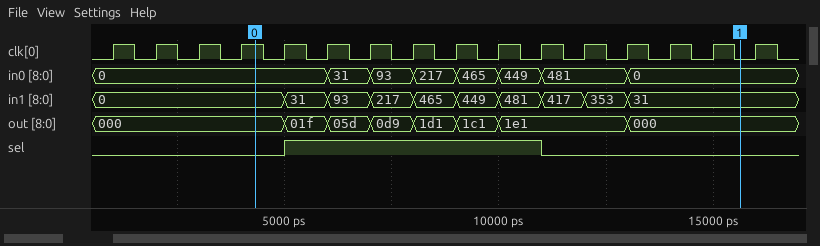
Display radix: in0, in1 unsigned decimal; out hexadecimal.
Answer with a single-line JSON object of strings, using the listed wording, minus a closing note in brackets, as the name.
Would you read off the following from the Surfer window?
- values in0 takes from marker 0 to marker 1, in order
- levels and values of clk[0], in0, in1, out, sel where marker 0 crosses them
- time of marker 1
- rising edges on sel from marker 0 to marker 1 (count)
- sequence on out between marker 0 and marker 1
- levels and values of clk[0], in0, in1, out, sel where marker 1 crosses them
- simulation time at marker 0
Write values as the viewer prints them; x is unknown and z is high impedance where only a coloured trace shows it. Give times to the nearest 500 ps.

{"values in0 takes from marker 0 to marker 1, in order": "0, 31, 93, 217, 465, 449, 481, 0", "levels and values of clk[0], in0, in1, out, sel where marker 0 crosses them": "clk[0]=1, in0=0, in1=0, out=000, sel=0", "time of marker 1": "15500 ps", "rising edges on sel from marker 0 to marker 1": "1", "sequence on out between marker 0 and marker 1": "000, 01f, 05d, 0d9, 1d1, 1c1, 1e1, 000", "levels and values of clk[0], in0, in1, out, sel where marker 1 crosses them": "clk[0]=0, in0=0, in1=31, out=000, sel=0", "simulation time at marker 0": "4500 ps"}
